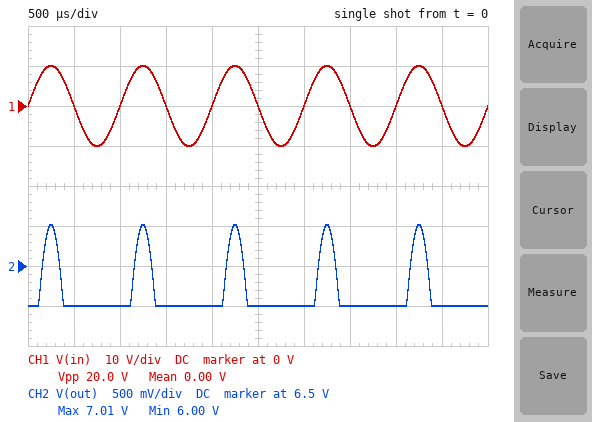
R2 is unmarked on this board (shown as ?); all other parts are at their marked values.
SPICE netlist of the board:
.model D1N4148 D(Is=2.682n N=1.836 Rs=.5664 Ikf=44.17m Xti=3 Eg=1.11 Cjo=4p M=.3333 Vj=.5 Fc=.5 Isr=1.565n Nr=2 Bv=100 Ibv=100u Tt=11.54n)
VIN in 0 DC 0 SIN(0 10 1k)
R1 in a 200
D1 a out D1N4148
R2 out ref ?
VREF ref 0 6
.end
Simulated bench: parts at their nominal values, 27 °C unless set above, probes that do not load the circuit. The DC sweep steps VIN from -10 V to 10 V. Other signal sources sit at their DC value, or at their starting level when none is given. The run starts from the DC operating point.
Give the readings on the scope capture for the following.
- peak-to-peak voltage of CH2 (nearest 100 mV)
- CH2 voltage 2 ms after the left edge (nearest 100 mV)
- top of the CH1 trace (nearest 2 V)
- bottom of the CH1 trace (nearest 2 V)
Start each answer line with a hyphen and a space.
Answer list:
- 1.0 V
- 6.0 V
- 10 V
- -10 V
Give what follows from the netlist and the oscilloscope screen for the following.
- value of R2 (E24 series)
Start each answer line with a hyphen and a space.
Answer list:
- 91 Ω
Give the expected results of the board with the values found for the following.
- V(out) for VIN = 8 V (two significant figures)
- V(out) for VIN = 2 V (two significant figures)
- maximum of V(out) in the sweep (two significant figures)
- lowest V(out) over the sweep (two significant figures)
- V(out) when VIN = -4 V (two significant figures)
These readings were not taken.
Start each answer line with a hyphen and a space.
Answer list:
- 6.4 V
- 6.0 V
- 7.0 V
- 6.0 V
- 6.0 V
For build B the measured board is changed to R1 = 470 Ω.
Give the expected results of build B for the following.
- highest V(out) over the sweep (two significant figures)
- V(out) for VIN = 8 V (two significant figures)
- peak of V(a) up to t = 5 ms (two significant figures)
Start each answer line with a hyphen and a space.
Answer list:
- 6.5 V
- 6.2 V
- 7.2 V
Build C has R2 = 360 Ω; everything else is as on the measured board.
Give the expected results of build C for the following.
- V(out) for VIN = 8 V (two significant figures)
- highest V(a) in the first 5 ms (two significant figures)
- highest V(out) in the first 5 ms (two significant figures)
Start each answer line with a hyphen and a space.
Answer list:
- 6.9 V
- 8.8 V
- 8.1 V
